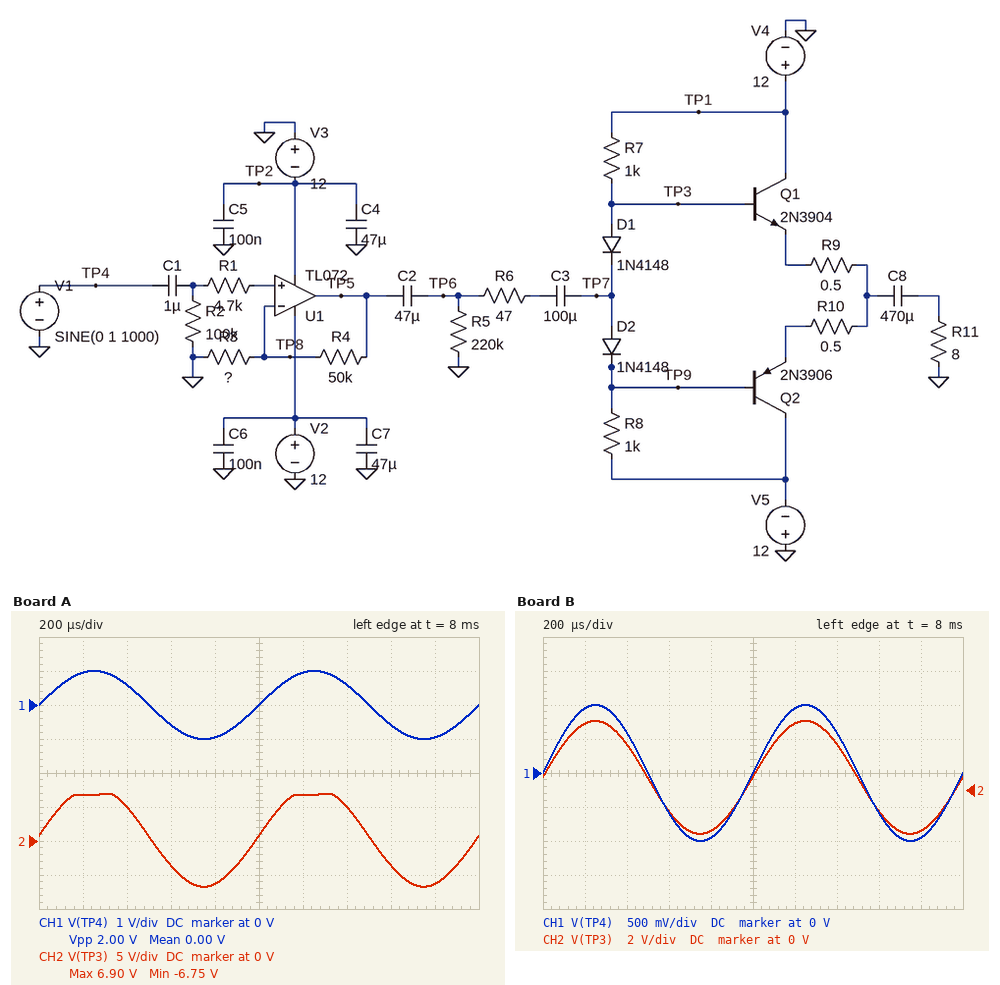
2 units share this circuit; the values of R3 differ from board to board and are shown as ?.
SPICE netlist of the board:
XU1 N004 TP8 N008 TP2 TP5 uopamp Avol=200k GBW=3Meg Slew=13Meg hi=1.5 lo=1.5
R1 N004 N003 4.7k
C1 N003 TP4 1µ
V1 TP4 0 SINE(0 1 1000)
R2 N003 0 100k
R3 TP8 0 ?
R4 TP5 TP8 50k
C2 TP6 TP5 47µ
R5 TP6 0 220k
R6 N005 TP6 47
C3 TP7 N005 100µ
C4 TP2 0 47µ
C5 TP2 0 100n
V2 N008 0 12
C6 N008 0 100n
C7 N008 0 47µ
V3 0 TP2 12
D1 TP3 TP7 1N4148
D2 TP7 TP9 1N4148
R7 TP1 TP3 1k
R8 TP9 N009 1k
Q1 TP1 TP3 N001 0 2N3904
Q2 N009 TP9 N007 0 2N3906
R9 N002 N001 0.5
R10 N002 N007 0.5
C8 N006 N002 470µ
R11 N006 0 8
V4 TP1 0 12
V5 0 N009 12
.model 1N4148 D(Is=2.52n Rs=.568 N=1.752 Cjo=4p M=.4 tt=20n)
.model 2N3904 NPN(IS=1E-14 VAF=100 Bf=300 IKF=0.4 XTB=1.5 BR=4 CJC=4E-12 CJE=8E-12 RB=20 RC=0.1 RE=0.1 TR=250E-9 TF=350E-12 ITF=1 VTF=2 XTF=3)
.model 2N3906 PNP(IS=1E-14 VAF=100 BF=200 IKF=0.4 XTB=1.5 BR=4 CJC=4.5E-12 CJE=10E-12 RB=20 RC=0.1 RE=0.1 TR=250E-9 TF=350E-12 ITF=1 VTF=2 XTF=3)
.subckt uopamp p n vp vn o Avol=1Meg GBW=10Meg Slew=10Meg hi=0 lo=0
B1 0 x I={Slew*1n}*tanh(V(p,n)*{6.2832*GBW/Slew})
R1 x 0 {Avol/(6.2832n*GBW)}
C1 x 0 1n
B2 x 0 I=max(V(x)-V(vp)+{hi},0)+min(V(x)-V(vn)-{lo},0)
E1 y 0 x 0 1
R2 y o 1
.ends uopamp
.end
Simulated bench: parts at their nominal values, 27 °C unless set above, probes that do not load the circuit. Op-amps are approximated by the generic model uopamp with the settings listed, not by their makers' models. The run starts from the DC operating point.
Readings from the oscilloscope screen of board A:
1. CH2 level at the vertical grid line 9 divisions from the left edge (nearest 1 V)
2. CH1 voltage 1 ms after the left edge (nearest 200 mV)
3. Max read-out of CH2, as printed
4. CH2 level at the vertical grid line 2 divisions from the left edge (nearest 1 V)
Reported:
-6 V
0 V
6.90 V
5 V
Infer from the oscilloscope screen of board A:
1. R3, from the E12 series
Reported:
6.8 kΩ
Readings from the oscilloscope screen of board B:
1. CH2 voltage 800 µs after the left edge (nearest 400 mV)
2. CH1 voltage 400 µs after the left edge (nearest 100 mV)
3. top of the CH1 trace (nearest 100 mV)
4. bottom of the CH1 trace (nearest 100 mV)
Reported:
-2.4 V
600 mV
1.0 V
-1.0 V
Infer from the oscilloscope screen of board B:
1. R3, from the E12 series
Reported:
18 kΩ
